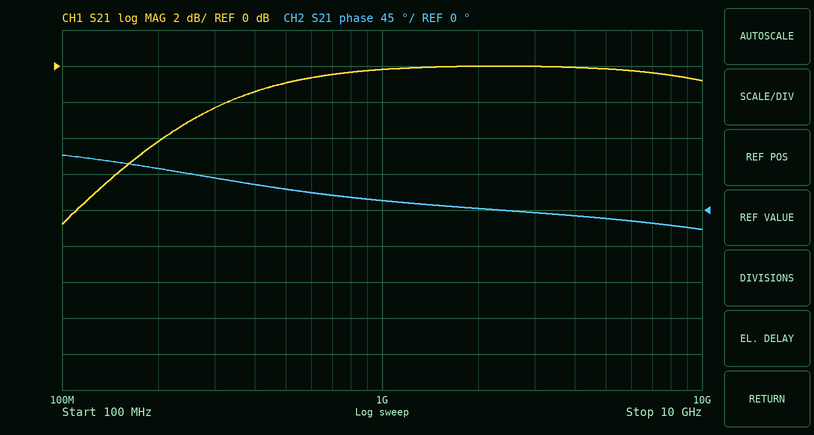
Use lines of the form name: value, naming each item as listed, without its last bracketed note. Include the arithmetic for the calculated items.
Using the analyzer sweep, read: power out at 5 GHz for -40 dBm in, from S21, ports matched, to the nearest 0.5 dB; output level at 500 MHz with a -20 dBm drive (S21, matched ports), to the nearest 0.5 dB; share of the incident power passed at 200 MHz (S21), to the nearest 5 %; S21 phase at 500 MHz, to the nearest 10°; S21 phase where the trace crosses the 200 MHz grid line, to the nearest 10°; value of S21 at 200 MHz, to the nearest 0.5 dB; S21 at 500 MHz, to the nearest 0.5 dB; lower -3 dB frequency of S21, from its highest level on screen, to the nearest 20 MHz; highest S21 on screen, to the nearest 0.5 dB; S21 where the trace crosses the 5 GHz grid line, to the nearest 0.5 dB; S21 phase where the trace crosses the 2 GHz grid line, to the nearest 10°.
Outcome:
power out at 5 GHz for -40 dBm in, from S21, ports matched, to the nearest 0.5 dB: -40 dBm + (0.0 dB) = -40.0 dBm
output level at 500 MHz with a -20 dBm drive (S21, matched ports), to the nearest 0.5 dB: -20 dBm + (-1.0 dB) = -21.0 dBm
share of the incident power passed at 200 MHz (S21), to the nearest 5 %: 10^(-4/10) ≈ 40 %
S21 phase at 500 MHz, to the nearest 10°: 30°
S21 phase where the trace crosses the 200 MHz grid line, to the nearest 10°: 50°
value of S21 at 200 MHz, to the nearest 0.5 dB: -4.0 dB
S21 at 500 MHz, to the nearest 0.5 dB: -1.0 dB
lower -3 dB frequency of S21, from its highest level on screen, to the nearest 20 MHz: 260 MHz
highest S21 on screen, to the nearest 0.5 dB: 0.0 dB
S21 where the trace crosses the 5 GHz grid line, to the nearest 0.5 dB: 0.0 dB
S21 phase where the trace crosses the 2 GHz grid line, to the nearest 10°: 0°
